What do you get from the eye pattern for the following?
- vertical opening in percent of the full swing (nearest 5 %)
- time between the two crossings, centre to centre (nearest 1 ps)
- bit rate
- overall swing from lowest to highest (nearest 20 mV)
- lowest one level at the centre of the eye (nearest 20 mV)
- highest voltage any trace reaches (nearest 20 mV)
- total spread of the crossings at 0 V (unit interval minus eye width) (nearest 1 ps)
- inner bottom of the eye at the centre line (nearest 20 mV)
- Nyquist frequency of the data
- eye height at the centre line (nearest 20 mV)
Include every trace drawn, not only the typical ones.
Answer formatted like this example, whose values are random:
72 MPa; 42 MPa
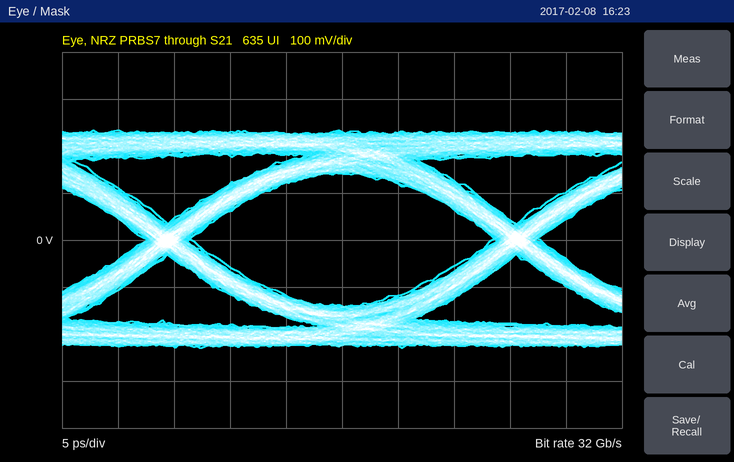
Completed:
60 %; 31 ps; 32 Gb/s; 460 mV; 140 mV; 240 mV; 4 ps; -140 mV; 16 GHz; 280 mV
